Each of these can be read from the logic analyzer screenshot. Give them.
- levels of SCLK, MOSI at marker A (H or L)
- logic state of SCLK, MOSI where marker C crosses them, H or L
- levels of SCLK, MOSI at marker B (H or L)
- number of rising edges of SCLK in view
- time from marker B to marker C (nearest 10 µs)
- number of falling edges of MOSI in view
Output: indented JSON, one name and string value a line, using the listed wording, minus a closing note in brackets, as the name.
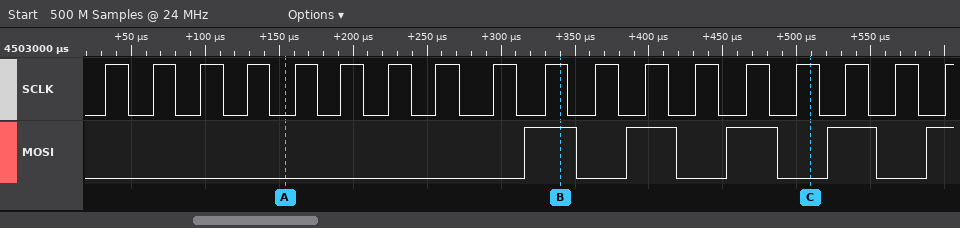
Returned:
{
  "levels of SCLK, MOSI at marker A": "SCLK=L, MOSI=L",
  "logic state of SCLK, MOSI where marker C crosses them, H or L": "SCLK=H, MOSI=L",
  "levels of SCLK, MOSI at marker B": "SCLK=H, MOSI=H",
  "number of rising edges of SCLK in view": "18",
  "time from marker B to marker C": "170 µs",
  "number of falling edges of MOSI in view": "4"
}
